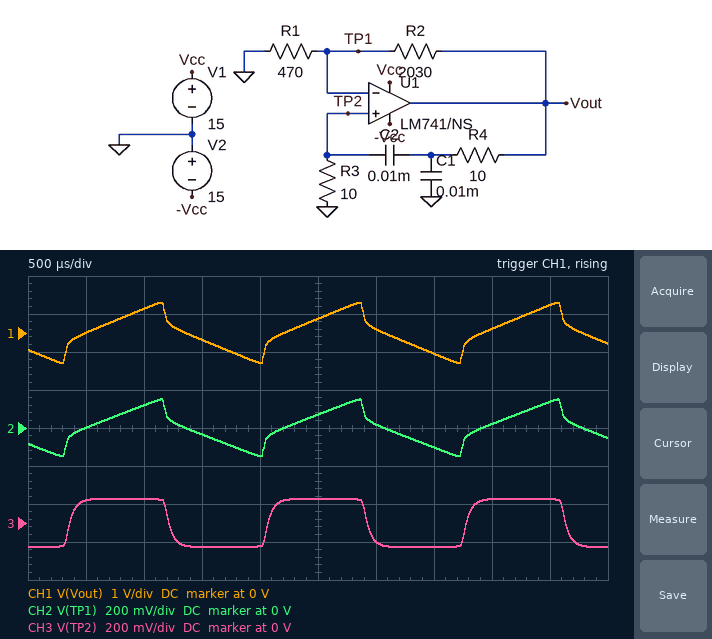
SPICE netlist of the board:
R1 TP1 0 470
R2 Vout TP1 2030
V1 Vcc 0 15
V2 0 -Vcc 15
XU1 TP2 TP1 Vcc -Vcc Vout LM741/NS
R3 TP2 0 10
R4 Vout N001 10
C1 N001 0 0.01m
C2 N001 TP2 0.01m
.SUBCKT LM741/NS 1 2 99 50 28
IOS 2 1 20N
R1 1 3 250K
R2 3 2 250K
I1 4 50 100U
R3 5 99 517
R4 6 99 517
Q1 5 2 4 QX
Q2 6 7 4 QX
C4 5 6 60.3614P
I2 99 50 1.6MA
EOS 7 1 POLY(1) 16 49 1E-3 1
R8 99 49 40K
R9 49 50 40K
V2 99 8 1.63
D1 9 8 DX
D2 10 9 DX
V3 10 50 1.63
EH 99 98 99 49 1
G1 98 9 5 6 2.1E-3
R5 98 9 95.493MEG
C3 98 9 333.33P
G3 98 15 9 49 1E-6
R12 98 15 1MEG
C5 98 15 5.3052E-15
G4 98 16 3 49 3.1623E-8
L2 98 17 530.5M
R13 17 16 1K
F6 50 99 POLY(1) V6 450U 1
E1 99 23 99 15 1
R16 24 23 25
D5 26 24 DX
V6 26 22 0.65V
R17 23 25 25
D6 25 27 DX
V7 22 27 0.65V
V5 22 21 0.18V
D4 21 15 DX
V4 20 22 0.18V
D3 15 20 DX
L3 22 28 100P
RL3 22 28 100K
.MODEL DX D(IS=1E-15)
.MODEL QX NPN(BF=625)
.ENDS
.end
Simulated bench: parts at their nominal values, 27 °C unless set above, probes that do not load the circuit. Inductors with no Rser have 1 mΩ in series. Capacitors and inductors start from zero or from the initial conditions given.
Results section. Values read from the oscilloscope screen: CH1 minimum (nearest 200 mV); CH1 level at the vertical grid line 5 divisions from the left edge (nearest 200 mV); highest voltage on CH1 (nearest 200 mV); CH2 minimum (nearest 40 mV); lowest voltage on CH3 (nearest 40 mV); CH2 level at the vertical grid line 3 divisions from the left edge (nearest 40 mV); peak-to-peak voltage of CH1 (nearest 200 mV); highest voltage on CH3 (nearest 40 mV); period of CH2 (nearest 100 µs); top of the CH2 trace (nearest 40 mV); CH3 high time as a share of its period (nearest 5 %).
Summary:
-800 mV
400 mV
800 mV
-160 mV
-120 mV
-40 mV
1.6 V
120 mV
1.7 ms
160 mV
50 %
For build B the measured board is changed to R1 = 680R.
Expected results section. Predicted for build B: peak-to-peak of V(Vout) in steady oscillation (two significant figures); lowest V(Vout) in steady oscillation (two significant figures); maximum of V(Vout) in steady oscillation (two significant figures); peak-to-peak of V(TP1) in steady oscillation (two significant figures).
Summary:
1.2 V
-610 mV
620 mV
310 mV
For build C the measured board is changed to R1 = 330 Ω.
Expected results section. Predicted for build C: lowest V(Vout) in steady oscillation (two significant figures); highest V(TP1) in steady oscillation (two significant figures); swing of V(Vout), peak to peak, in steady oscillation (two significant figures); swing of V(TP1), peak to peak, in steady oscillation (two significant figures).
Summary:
-1.0 V
150 mV
2.1 V
290 mV
